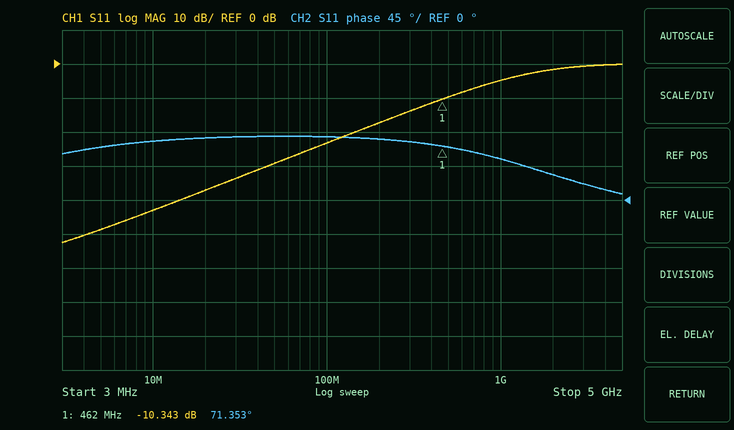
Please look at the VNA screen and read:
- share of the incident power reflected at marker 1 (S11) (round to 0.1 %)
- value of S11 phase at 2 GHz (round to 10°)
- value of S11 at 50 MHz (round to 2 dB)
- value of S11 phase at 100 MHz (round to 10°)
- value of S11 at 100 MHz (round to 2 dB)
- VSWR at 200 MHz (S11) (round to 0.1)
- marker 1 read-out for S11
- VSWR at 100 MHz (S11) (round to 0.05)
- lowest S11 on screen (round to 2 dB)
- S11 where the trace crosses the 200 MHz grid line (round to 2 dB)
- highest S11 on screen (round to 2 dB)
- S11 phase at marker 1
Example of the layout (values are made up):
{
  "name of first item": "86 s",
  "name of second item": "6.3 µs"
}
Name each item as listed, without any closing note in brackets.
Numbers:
{
  "share of the incident power reflected at marker 1 (S11)": "9.2 %",
  "value of S11 phase at 2 GHz": "30°",
  "value of S11 at 50 MHz": "-30 dB",
  "value of S11 phase at 100 MHz": "80°",
  "value of S11 at 100 MHz": "-24 dB",
  "VSWR at 200 MHz (S11)": "1.3",
  "marker 1 read-out for S11": "-10.343 dB",
  "VSWR at 100 MHz (S11)": "1.15",
  "lowest S11 on screen": "-52 dB",
  "S11 where the trace crosses the 200 MHz grid line": "-18 dB",
  "highest S11 on screen": "0 dB",
  "S11 phase at marker 1": "71.353°"
}
